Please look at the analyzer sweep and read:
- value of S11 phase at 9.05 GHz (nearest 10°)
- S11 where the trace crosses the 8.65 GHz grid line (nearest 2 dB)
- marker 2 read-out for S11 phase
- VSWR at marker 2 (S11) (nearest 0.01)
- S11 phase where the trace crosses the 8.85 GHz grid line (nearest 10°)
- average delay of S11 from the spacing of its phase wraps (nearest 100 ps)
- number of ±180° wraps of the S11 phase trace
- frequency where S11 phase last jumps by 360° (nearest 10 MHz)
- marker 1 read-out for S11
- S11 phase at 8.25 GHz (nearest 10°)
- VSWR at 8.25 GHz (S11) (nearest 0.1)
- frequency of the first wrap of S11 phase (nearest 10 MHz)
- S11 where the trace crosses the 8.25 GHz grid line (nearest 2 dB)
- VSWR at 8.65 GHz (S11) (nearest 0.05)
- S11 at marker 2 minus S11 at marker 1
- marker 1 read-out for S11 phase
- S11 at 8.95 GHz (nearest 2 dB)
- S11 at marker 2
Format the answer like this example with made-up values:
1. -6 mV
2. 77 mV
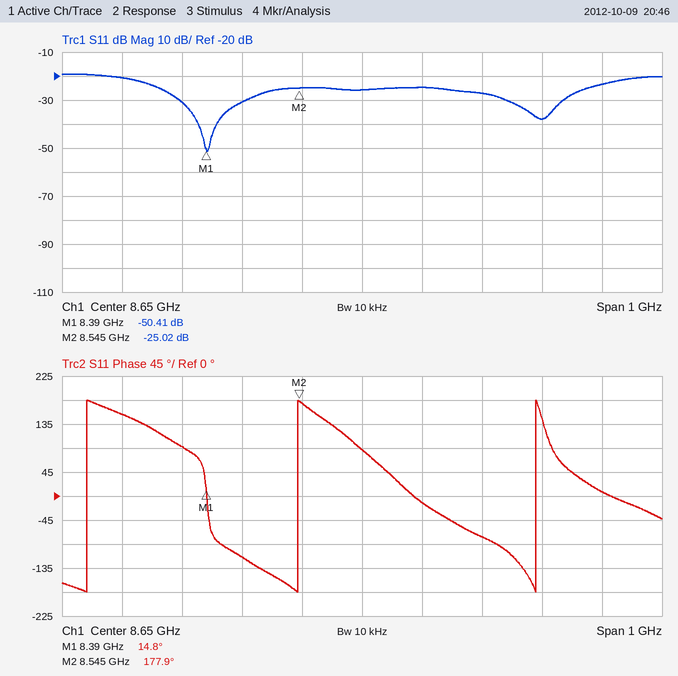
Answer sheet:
1. 10°
2. -26 dB
3. 177.9°
4. 1.12
5. -80°
6. 2.7 ns
7. 3
8. 8.94 GHz
9. -50.41 dB
10. 150°
11. 1.2
12. 8.19 GHz
13. -20 dB
14. 1.10
15. 25.39 dB
16. 14.8°
17. -38 dB
18. -25.02 dB
